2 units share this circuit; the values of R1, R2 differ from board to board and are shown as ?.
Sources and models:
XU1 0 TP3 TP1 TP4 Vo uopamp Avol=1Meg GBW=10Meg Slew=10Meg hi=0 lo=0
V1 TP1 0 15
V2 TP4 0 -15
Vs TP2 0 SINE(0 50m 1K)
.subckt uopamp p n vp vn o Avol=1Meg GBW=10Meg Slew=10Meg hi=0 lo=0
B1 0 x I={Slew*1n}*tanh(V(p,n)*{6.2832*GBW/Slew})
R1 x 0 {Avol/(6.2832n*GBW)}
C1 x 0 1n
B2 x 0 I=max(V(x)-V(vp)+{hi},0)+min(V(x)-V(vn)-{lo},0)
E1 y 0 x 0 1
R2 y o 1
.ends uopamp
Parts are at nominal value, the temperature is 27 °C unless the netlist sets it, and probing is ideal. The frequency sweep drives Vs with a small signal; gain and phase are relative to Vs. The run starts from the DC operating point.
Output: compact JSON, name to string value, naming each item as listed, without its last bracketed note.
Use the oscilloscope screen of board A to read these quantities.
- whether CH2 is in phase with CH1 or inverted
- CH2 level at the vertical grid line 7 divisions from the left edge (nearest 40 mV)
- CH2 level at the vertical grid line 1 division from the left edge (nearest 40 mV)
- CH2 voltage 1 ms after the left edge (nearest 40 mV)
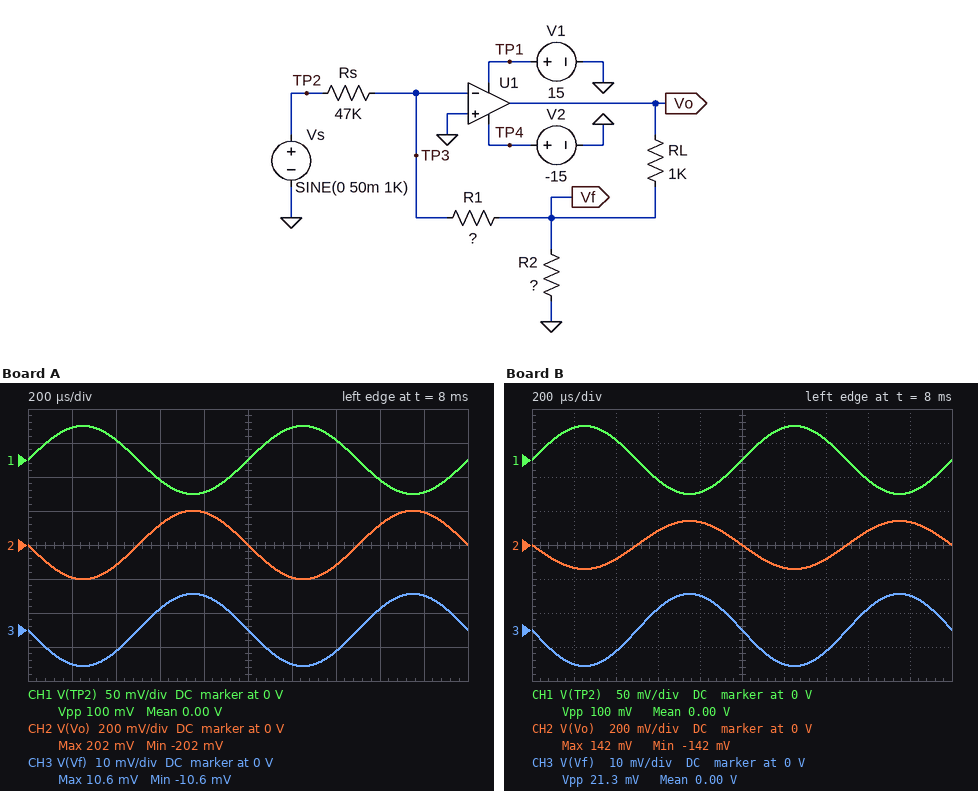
{"whether CH2 is in phase with CH1 or inverted": "inverted", "CH2 level at the vertical grid line 7 divisions from the left edge": "-120 mV", "CH2 level at the vertical grid line 1 division from the left edge": "-200 mV", "CH2 voltage 1 ms after the left edge": "0 V"}
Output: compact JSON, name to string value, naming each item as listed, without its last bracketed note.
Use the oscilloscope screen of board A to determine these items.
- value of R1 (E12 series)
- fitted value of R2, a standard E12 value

{"value of R1": "10 kΩ", "fitted value of R2, a standard E12 value": "56 Ω"}
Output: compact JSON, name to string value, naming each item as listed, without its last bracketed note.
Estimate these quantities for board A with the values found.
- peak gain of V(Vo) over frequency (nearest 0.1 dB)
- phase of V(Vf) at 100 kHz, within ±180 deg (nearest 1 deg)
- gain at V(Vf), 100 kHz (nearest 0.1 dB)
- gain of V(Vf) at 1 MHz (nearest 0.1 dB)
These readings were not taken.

{"peak gain of V(Vo) over frequency": "12.1 dB", "phase of V(Vf) at 100 kHz, within ±180 deg": "167 deg", "gain at V(Vf), 100 kHz": "-13.7 dB", "gain of V(Vf) at 1 MHz": "-21.4 dB"}
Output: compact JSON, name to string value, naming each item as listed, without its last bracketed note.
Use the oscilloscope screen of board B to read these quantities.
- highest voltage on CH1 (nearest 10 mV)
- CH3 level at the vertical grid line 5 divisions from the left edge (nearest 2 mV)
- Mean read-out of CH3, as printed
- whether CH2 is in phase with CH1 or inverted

{"highest voltage on CH1": "50 mV", "CH3 level at the vertical grid line 5 divisions from the left edge": "0 V", "Mean read-out of CH3, as printed": "0.00 V", "whether CH2 is in phase with CH1 or inverted": "inverted"}
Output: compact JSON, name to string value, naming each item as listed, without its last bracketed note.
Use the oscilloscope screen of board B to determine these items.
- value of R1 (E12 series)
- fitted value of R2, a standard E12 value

{"value of R1": "10 kΩ", "fitted value of R2, a standard E12 value": "82 Ω"}
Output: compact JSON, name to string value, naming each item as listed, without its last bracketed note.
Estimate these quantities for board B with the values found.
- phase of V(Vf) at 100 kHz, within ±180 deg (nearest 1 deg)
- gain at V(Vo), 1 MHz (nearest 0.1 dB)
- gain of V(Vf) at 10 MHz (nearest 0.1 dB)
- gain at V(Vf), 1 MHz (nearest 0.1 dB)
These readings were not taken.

{"phase of V(Vf) at 100 kHz, within ±180 deg": "171 deg", "gain at V(Vo), 1 MHz": "3.5 dB", "gain of V(Vf) at 10 MHz": "-37.5 dB", "gain at V(Vf), 1 MHz": "-19.0 dB"}
